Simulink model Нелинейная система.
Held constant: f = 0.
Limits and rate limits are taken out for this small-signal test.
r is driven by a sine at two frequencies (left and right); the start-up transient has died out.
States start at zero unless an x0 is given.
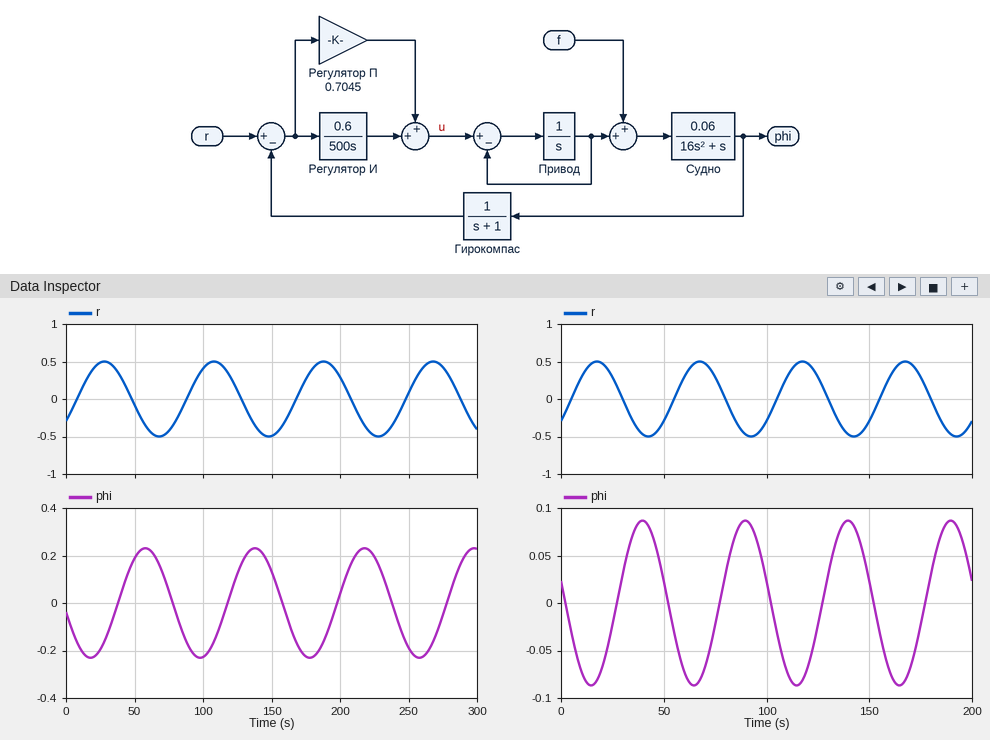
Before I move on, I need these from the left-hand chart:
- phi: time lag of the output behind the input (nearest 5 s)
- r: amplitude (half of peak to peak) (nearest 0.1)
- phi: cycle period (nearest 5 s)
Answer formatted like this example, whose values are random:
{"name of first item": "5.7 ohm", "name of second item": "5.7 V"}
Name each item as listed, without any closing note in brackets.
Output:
{"phi: time lag of the output behind the input": "30 s", "r: amplitude (half of peak to peak)": "0.5", "phi: cycle period": "80 s"}
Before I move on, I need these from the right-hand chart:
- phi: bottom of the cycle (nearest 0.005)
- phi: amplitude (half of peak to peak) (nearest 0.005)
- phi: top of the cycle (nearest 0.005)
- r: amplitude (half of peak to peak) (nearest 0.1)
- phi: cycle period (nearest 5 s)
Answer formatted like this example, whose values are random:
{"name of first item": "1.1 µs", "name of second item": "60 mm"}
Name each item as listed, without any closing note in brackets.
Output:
{"phi: bottom of the cycle": "-0.085", "phi: amplitude (half of peak to peak)": "0.085", "phi: top of the cycle": "0.085", "r: amplitude (half of peak to peak)": "0.5", "phi: cycle period": "50 s"}
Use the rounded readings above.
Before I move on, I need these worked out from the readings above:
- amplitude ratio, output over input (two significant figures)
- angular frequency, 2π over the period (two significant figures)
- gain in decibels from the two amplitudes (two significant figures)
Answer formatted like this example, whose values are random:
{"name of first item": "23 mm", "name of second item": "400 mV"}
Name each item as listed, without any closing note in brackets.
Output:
{"amplitude ratio, output over input": "0.17", "angular frequency, 2π over the period": "0.13 rad/s", "gain in decibels from the two amplitudes": "-15 dB"}
